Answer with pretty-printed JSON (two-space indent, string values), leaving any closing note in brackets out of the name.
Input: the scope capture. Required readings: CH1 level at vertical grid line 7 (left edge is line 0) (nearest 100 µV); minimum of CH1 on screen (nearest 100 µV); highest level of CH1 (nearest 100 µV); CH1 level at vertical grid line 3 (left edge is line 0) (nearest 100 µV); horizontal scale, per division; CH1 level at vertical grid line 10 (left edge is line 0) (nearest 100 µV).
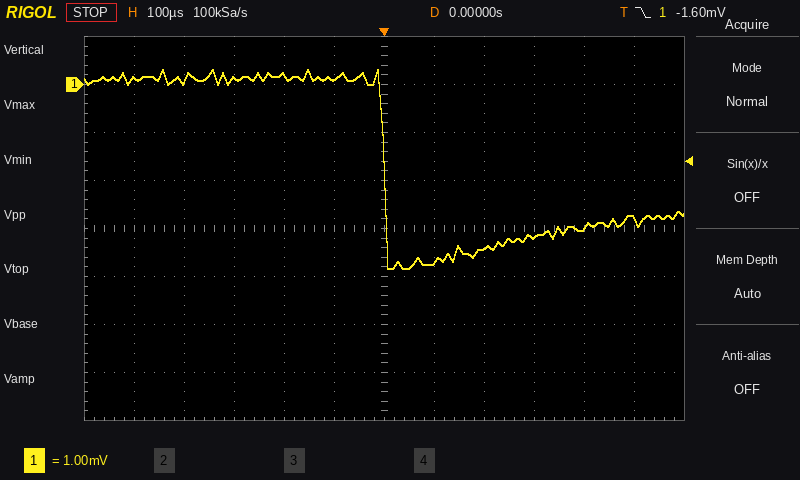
{
  "CH1 level at vertical grid line 7 (left edge is line 0)": "-3.7 mV",
  "minimum of CH1 on screen": "-3.8 mV",
  "highest level of CH1": "300 µV",
  "CH1 level at vertical grid line 3 (left edge is line 0)": "100 µV",
  "horizontal scale, per division": "100 µs",
  "CH1 level at vertical grid line 10 (left edge is line 0)": "-3.0 mV"
}
